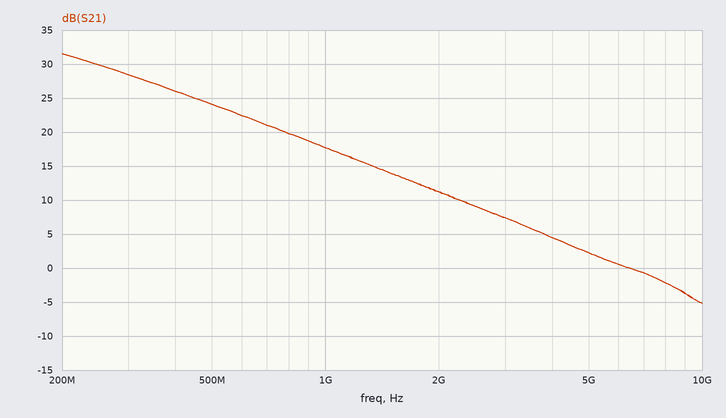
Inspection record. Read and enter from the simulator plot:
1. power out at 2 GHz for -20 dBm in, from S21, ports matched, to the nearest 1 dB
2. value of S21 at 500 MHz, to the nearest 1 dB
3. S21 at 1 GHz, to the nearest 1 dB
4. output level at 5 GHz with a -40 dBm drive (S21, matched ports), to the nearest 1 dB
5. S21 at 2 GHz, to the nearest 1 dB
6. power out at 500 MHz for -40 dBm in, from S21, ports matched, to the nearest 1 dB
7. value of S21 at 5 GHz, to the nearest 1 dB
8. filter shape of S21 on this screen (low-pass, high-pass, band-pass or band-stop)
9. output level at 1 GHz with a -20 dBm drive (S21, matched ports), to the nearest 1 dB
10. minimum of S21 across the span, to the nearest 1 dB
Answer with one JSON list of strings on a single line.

["-9 dBm", "24 dB", "18 dB", "-38 dBm", "11 dB", "-16 dBm", "2 dB", "low-pass", "-2 dBm", "-5 dB"]
